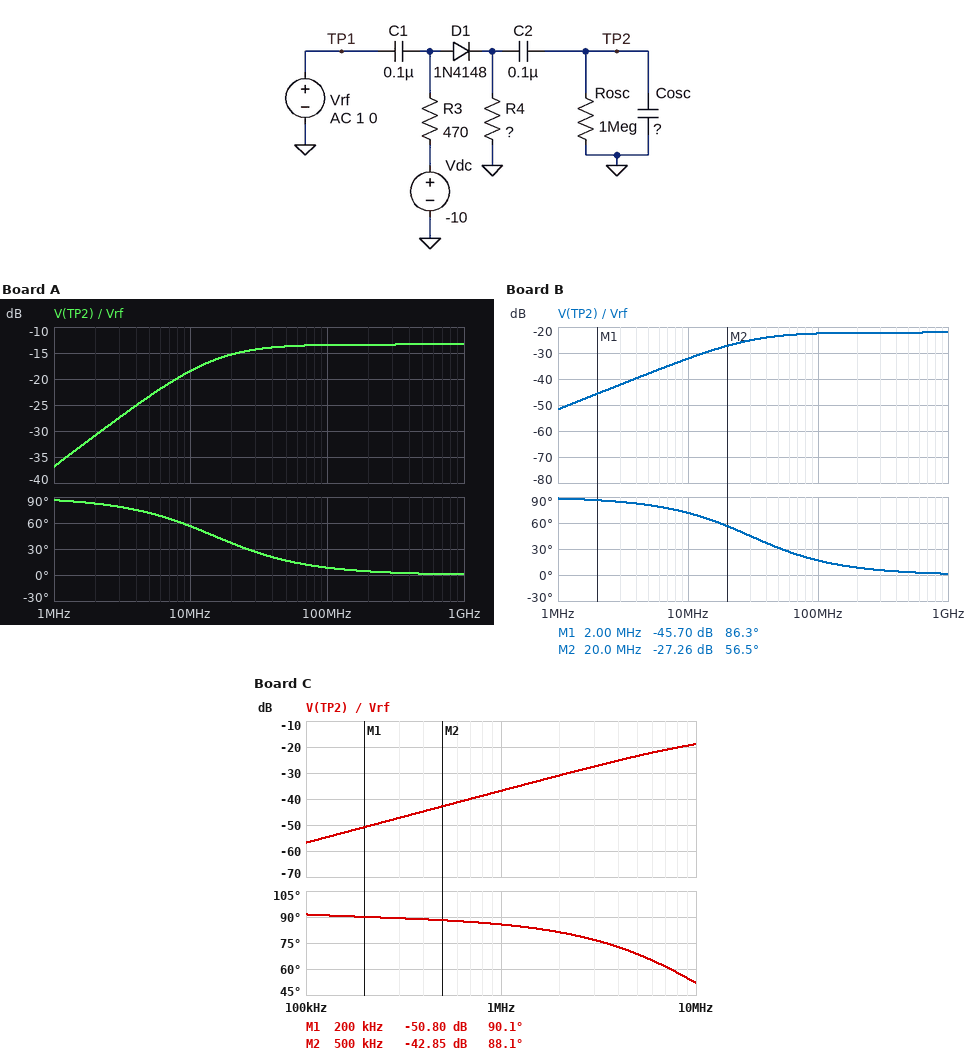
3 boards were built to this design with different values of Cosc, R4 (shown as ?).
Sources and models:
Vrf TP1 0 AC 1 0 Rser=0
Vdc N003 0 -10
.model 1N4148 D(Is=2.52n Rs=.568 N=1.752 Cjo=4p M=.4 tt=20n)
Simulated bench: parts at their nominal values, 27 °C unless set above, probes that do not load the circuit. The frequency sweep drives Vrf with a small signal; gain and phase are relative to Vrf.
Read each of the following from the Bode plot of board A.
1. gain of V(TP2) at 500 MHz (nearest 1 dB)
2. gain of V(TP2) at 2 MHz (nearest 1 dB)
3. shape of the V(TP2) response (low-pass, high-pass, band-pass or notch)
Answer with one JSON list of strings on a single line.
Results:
["-13 dB", "-31 dB", "high-pass"]
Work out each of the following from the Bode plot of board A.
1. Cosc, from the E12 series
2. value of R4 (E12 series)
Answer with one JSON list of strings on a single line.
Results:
["5.6 pF", "1.5 kΩ"]
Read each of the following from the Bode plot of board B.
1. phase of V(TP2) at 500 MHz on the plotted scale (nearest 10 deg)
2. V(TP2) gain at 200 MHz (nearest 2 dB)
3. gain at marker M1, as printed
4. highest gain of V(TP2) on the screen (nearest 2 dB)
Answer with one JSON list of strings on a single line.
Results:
["0 deg", "-22 dB", "-45.70 dB", "-22 dB"]
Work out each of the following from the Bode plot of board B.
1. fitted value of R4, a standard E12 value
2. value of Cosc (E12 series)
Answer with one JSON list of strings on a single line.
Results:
["270 Ω", "18 pF"]
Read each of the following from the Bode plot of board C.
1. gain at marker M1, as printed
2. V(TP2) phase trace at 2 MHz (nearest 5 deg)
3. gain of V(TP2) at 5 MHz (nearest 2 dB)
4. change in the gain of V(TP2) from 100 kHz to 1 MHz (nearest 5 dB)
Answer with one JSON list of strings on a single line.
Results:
["-50.80 dB", "80 deg", "-24 dB", "20 dB"]
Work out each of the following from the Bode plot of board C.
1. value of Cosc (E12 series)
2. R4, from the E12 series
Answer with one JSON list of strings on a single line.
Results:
["6.8 pF", "1.5 kΩ"]
